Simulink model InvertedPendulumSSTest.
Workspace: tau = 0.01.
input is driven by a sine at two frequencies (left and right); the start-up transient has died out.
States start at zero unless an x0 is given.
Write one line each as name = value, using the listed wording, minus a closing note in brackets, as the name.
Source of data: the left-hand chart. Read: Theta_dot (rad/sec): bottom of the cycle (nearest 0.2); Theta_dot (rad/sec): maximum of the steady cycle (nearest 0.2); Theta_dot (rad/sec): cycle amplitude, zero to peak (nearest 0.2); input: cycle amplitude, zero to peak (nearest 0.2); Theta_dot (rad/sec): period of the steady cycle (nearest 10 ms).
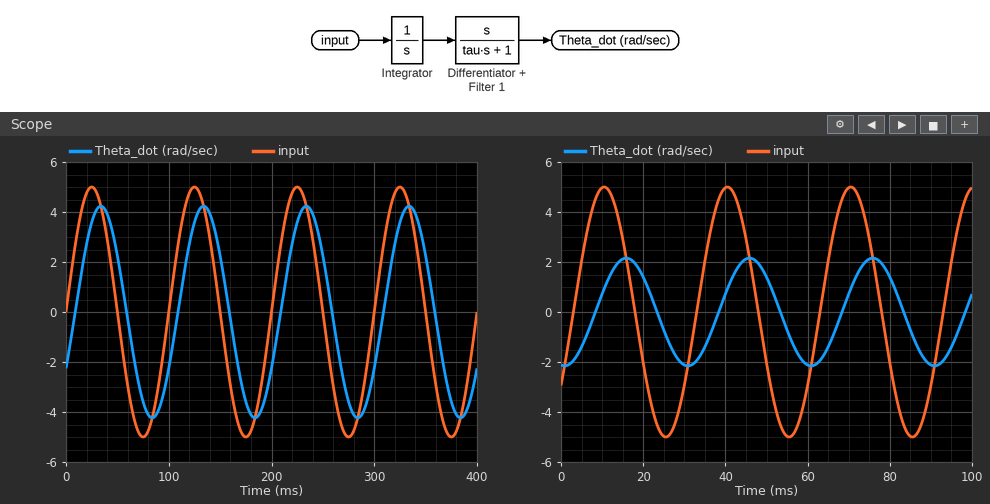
Theta_dot (rad/sec): bottom of the cycle = -4.2
Theta_dot (rad/sec): maximum of the steady cycle = 4.2
Theta_dot (rad/sec): cycle amplitude, zero to peak = 4.2
input: cycle amplitude, zero to peak = 5.0
Theta_dot (rad/sec): period of the steady cycle = 100 ms
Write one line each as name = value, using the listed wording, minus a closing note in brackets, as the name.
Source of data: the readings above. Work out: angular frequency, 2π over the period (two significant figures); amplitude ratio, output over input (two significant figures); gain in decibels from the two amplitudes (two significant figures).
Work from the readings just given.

angular frequency, 2π over the period = 0.063 rad/ms
amplitude ratio, output over input = 0.84
gain in decibels from the two amplitudes = -1.5 dB
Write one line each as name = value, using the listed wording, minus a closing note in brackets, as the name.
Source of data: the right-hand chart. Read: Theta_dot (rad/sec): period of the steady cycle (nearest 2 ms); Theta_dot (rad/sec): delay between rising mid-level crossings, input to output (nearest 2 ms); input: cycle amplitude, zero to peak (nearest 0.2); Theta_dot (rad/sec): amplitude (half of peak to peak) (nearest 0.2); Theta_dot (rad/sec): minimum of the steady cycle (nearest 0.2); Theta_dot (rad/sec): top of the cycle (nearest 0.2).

Theta_dot (rad/sec): period of the steady cycle = 30 ms
Theta_dot (rad/sec): delay between rising mid-level crossings, input to output = 6 ms
input: cycle amplitude, zero to peak = 5.0
Theta_dot (rad/sec): amplitude (half of peak to peak) = 2.2
Theta_dot (rad/sec): minimum of the steady cycle = -2.2
Theta_dot (rad/sec): top of the cycle = 2.2
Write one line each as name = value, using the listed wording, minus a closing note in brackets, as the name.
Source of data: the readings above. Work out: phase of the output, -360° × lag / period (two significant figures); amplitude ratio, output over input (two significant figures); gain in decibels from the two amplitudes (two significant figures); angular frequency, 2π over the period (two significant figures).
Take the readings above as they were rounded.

phase of the output, -360° × lag / period = -72°
amplitude ratio, output over input = 0.44
gain in decibels from the two amplitudes = -7.1 dB
angular frequency, 2π over the period = 0.21 rad/ms
